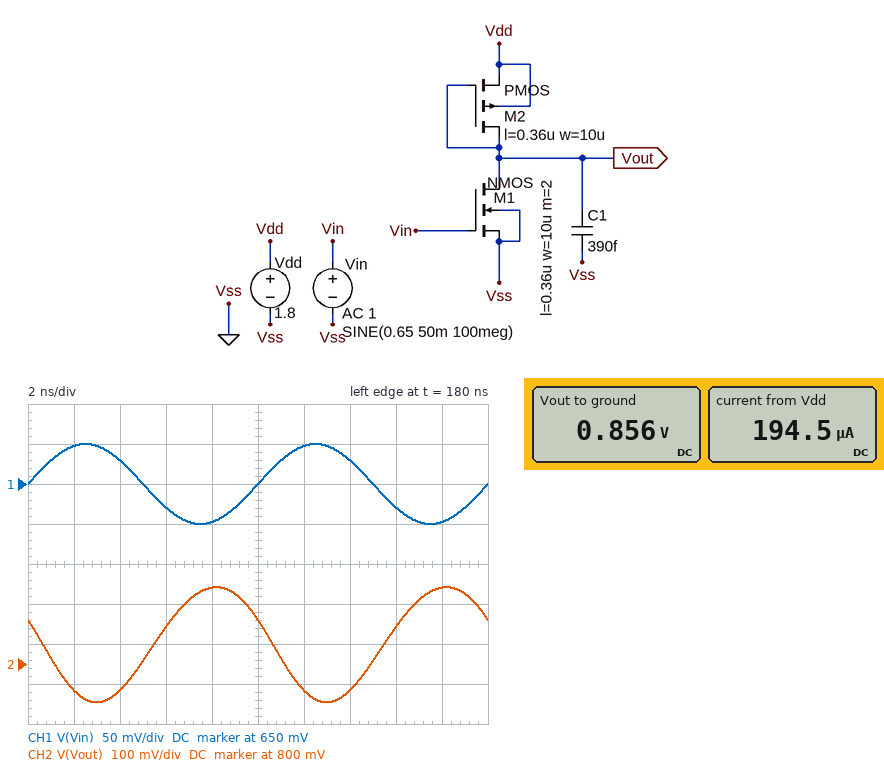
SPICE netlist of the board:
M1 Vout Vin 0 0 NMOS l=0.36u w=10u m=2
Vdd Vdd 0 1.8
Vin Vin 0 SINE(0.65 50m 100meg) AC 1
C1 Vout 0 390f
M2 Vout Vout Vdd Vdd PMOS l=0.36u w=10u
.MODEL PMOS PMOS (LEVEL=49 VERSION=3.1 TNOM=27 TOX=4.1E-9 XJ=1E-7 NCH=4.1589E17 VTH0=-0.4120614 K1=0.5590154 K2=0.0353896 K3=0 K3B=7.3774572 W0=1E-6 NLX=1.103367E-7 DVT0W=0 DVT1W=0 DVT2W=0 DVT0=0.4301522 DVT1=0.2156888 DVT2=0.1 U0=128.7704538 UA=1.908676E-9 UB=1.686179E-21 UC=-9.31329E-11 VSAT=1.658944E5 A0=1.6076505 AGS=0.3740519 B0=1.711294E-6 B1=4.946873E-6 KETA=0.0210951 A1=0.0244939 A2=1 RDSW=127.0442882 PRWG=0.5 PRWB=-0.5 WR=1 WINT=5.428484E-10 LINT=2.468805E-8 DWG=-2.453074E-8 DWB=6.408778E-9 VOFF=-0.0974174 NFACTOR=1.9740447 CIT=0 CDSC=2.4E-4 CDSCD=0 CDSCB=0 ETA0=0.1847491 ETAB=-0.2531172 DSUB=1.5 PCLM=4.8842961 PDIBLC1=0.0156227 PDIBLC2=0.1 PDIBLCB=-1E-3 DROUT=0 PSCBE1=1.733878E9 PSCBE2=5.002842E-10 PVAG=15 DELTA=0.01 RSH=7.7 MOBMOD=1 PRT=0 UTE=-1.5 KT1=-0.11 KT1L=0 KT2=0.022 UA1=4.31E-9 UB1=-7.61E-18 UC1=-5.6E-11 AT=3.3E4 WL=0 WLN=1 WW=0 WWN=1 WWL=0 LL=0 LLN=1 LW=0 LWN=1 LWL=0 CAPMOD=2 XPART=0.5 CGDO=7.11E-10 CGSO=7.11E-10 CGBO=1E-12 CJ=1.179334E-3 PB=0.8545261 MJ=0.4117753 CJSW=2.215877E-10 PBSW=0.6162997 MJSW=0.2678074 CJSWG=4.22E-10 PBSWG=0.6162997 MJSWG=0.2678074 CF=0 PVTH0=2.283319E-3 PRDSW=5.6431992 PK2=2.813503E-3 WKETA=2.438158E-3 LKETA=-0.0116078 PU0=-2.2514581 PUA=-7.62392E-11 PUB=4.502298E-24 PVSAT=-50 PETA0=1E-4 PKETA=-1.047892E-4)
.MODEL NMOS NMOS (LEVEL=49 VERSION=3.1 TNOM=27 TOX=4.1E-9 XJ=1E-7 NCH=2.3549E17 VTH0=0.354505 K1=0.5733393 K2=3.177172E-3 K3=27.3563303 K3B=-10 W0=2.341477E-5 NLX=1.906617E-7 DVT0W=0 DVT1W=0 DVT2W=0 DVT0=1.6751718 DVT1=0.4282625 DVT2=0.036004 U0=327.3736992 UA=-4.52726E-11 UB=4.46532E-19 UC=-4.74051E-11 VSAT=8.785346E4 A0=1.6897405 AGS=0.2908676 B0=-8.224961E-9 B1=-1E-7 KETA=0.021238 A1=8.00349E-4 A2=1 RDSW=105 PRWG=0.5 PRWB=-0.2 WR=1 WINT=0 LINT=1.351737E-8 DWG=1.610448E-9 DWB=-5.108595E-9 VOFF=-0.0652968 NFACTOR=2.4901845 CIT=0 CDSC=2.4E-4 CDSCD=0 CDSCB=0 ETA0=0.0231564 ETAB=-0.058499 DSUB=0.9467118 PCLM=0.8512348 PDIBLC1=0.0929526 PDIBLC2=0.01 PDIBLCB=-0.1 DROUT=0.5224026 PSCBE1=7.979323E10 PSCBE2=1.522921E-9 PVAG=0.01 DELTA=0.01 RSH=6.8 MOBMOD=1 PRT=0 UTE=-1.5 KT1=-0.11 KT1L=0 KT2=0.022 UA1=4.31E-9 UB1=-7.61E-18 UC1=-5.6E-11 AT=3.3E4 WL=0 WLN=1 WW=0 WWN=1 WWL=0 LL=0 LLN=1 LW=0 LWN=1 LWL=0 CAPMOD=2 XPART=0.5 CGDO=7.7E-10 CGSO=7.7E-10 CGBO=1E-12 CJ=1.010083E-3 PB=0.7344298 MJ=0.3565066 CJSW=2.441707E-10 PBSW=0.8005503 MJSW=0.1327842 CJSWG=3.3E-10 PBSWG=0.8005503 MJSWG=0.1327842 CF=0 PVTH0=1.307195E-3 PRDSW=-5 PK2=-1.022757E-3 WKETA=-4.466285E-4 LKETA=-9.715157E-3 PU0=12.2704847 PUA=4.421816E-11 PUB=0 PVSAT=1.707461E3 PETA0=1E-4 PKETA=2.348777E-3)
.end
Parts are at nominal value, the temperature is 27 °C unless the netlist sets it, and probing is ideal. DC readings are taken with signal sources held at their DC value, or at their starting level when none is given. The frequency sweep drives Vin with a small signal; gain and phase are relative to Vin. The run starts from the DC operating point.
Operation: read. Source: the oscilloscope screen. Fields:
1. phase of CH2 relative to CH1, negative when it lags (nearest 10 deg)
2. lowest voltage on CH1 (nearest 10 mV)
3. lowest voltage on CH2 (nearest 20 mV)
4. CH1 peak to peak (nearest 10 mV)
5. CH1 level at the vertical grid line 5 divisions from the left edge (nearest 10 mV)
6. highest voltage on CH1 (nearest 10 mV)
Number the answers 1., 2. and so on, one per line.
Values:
1. 160 deg
2. 600 mV
3. 700 mV
4. 100 mV
5. 650 mV
6. 700 mV
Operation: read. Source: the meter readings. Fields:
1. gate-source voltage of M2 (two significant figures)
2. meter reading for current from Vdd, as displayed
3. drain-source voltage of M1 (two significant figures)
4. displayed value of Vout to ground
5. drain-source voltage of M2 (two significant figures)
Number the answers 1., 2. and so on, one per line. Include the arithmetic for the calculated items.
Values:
1. 856 mV - 1.8 V = -940 mV
2. 194.5 µA
3. 856 mV = 860 mV
4. 0.856 V
5. 856 mV - 1.8 V = -940 mV
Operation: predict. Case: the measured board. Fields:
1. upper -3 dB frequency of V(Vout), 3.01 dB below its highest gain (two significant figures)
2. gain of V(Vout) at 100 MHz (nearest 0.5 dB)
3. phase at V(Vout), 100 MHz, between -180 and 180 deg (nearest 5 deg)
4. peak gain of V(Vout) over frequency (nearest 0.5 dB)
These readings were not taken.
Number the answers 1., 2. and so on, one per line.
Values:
1. 280 MHz
2. 9.5 dB
3. 160 deg
4. 10.0 dB
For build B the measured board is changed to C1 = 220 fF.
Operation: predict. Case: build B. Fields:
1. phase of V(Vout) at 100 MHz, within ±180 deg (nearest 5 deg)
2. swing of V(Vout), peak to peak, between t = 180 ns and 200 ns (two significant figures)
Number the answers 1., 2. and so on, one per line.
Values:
1. 165 deg
2. 300 mV
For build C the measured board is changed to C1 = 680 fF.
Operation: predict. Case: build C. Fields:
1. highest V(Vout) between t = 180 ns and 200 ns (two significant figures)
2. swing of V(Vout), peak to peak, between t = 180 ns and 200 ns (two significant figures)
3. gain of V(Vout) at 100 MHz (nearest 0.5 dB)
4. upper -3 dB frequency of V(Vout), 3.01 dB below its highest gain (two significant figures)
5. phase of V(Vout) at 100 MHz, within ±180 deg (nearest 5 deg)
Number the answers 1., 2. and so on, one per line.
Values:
1. 980 mV
2. 260 mV
3. 8.5 dB
4. 170 MHz
5. 150 deg
